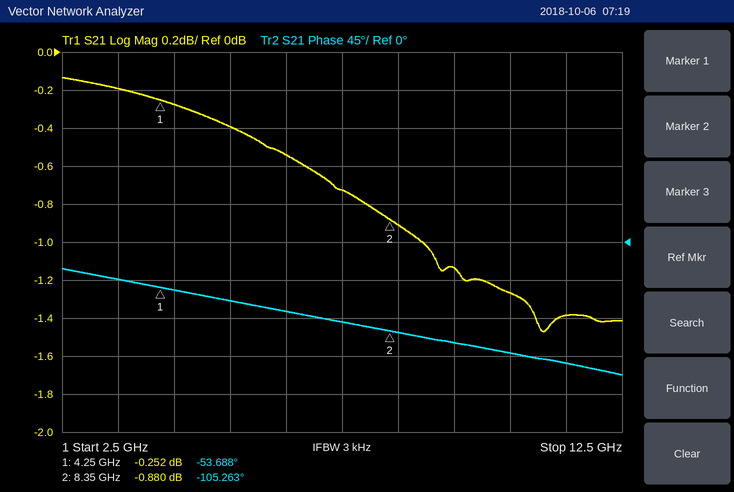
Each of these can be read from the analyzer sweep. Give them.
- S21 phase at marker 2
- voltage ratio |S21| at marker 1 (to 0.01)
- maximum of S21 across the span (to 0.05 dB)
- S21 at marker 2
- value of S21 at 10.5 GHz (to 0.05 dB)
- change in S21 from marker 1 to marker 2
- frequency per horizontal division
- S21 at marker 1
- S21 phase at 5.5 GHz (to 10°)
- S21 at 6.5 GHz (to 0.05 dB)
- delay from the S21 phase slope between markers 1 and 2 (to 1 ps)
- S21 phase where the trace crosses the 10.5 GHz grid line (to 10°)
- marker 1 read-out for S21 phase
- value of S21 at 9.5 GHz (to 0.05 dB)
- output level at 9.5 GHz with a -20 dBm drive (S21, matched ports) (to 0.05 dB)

-105.263°
0.97
-0.15 dB
-0.880 dB
-1.25 dB
-0.628 dB
1 GHz
-0.252 dB
-70°
-0.55 dB
35 ps
-130°
-53.688°
-1.15 dB
-21.15 dBm
